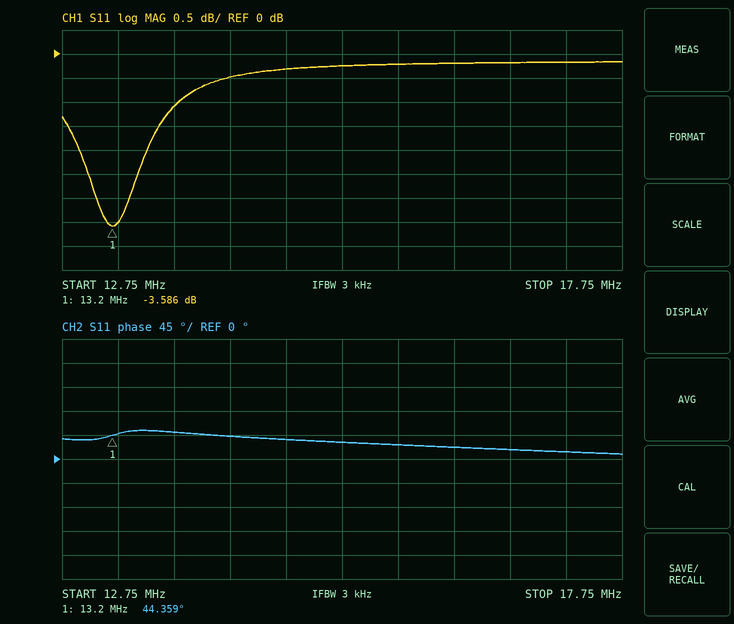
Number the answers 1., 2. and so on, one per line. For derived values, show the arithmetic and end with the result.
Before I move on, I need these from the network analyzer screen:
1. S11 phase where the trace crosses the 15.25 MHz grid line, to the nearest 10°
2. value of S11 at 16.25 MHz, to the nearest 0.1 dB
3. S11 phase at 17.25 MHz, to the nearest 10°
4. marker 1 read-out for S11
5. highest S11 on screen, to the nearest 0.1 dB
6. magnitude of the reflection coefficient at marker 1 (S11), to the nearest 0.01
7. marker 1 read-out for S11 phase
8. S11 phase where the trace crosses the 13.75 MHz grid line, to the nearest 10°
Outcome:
1. 30°
2. -0.2 dB
3. 10°
4. -3.586 dB
5. -0.2 dB
6. 10^(-3.586/20) ≈ 0.66
7. 44.359°
8. 50°
